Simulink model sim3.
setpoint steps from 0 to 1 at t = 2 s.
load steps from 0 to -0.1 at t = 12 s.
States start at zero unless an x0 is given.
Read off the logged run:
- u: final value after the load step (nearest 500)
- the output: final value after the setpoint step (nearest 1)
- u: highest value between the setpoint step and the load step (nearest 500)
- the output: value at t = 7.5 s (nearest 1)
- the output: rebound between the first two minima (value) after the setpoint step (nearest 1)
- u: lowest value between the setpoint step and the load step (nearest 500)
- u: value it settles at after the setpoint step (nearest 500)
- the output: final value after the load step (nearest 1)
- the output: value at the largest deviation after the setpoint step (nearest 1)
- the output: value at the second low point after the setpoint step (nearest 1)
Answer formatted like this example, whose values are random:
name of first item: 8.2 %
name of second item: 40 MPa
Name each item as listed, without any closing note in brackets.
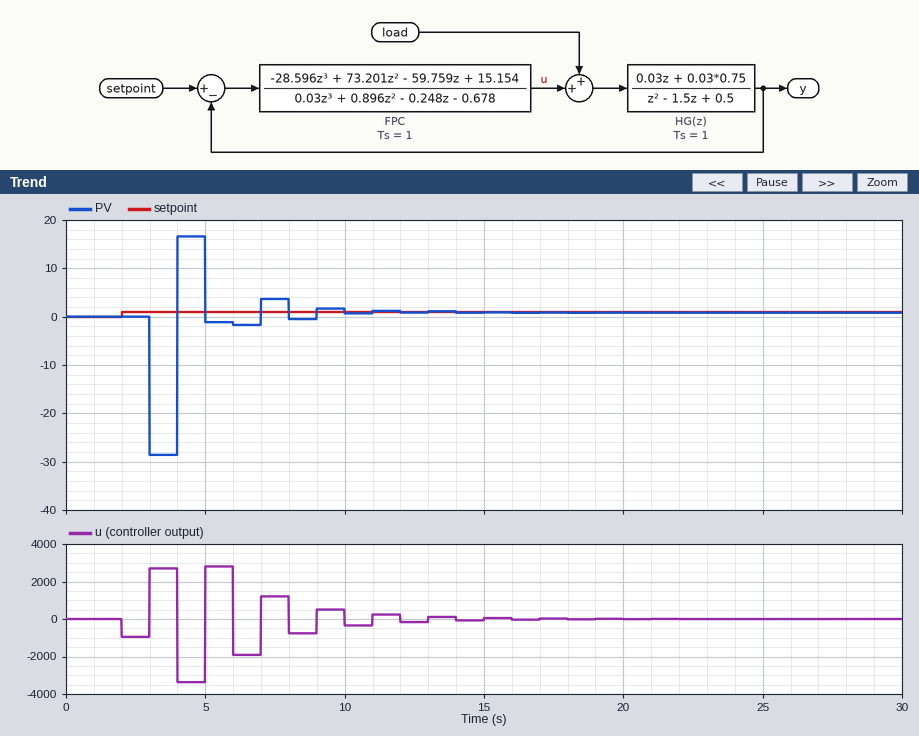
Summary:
u: final value after the load step: 0
the output: final value after the setpoint step: 1
u: highest value between the setpoint step and the load step: 3000
the output: value at t = 7.5 s: 4
the output: rebound between the first two minima (value) after the setpoint step: 17
u: lowest value between the setpoint step and the load step: -3500
u: value it settles at after the setpoint step: 0
the output: final value after the load step: 1
the output: value at the largest deviation after the setpoint step: -29
the output: value at the second low point after the setpoint step: -2
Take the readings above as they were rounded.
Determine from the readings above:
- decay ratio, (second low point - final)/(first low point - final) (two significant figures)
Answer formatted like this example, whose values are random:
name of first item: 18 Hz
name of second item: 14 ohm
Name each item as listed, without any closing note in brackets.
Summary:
decay ratio, (second low point - final)/(first low point - final): 0.10
